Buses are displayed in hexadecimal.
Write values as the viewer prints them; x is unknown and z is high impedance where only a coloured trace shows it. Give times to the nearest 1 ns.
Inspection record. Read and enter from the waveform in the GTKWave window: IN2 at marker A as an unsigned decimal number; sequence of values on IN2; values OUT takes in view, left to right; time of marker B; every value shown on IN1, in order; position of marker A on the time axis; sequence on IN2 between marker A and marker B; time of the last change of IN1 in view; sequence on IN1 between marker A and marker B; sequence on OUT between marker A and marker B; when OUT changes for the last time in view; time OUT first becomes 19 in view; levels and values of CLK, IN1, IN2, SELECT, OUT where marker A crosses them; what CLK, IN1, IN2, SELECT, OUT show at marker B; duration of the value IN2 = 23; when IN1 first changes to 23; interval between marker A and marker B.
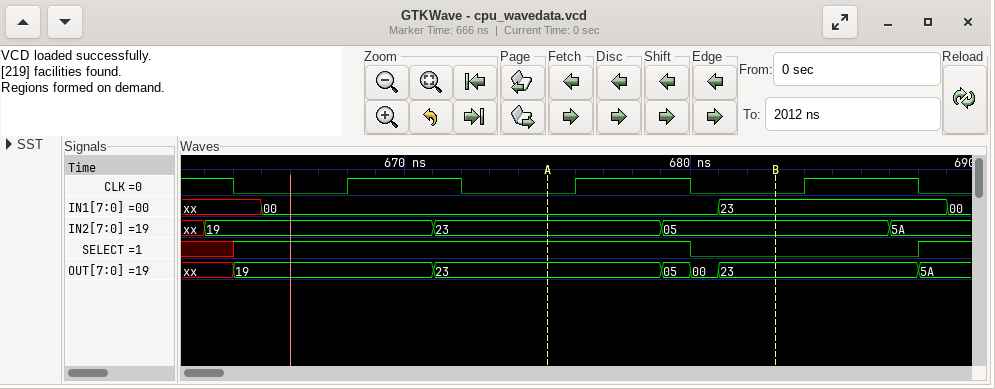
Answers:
35
xx, 19, 23, 05, 5A
xx, 19, 23, 05, 00, 23, 5A
683 ns
xx, 00, 23, 00
675 ns
23, 05
689 ns
00, 23
23, 05, 00, 23
688 ns
664 ns
CLK=0, IN1=00, IN2=23, SELECT=1, OUT=23
CLK=0, IN1=23, IN2=05, SELECT=0, OUT=23
8 ns
681 ns
8 ns
